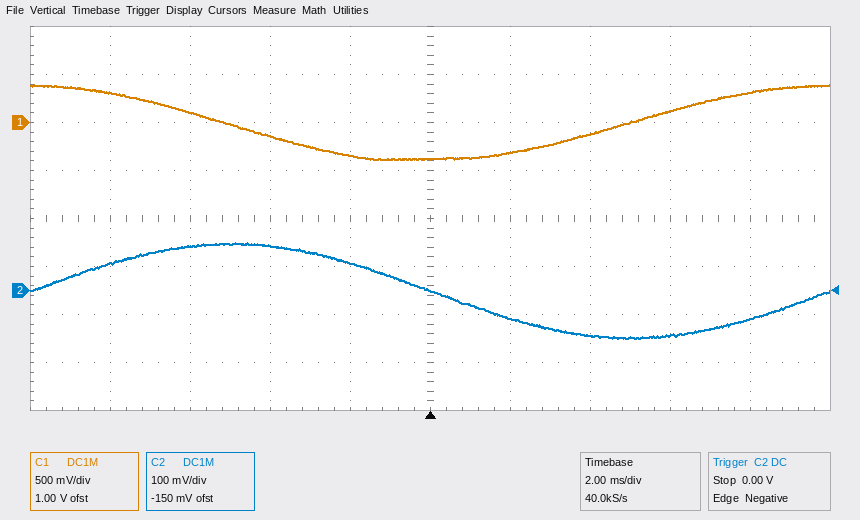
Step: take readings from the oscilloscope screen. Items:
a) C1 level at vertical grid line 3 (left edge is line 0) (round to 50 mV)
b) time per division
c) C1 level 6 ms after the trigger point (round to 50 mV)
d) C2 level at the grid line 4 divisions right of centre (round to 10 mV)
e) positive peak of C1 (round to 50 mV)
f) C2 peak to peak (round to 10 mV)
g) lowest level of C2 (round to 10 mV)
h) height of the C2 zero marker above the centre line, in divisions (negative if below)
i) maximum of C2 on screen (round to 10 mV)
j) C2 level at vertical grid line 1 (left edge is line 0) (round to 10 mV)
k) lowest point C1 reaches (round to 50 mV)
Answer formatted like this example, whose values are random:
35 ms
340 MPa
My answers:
-150 mV
2 ms
100 mV
-60 mV
400 mV
200 mV
-100 mV
-1.5 div
100 mV
60 mV
-400 mV
